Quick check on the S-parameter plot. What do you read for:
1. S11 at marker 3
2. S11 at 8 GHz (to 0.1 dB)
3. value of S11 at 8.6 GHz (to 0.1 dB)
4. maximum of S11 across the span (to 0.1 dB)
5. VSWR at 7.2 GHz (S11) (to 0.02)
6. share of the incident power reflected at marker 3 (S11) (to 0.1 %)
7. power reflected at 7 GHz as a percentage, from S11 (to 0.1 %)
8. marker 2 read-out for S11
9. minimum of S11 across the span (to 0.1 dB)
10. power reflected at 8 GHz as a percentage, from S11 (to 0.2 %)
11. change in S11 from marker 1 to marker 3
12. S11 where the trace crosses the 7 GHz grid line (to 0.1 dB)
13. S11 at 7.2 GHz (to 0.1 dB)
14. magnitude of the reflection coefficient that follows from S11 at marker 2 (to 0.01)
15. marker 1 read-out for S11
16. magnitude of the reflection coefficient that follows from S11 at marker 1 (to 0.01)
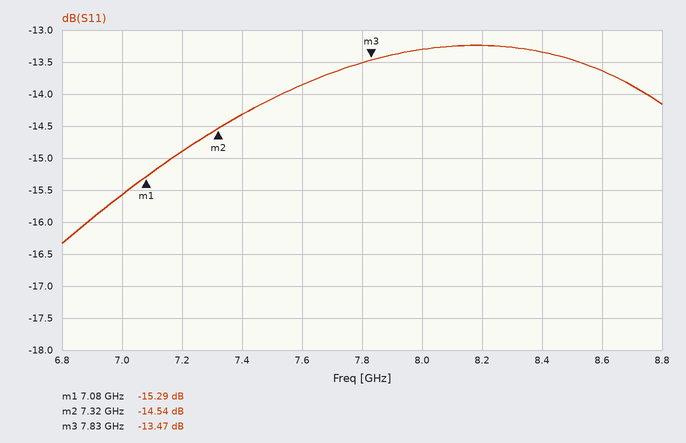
-13.47 dB
-13.3 dB
-13.6 dB
-13.2 dB
1.44
4.5 %
2.8 %
-14.54 dB
-16.3 dB
4.6 %
1.82 dB
-15.6 dB
-14.9 dB
0.19
-15.29 dB
0.17
